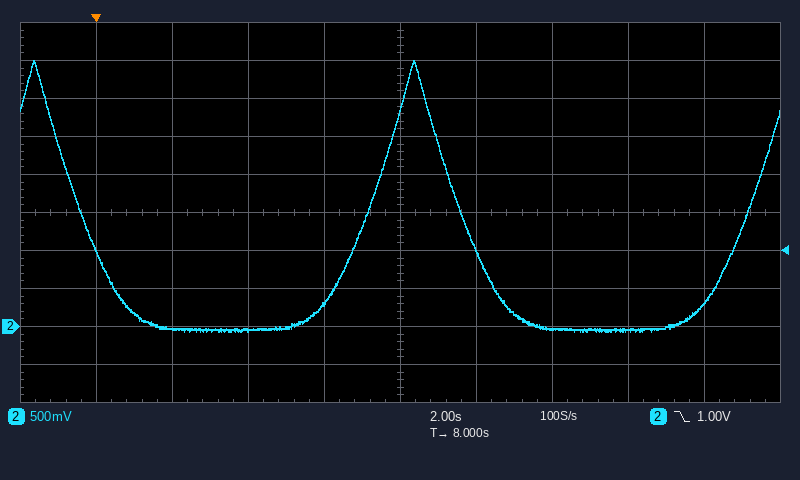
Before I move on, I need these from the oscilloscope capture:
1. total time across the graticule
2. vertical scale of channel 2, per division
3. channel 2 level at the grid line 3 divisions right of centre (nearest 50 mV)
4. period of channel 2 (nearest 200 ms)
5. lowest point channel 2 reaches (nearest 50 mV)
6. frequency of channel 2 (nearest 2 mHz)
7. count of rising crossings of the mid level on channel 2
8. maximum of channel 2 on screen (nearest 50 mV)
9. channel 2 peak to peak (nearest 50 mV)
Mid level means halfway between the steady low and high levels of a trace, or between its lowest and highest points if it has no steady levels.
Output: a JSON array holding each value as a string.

["20 s", "500 mV", "-50 mV", "10.0 s", "-50 mV", "100 mHz", "2", "3.50 V", "3.55 V"]
